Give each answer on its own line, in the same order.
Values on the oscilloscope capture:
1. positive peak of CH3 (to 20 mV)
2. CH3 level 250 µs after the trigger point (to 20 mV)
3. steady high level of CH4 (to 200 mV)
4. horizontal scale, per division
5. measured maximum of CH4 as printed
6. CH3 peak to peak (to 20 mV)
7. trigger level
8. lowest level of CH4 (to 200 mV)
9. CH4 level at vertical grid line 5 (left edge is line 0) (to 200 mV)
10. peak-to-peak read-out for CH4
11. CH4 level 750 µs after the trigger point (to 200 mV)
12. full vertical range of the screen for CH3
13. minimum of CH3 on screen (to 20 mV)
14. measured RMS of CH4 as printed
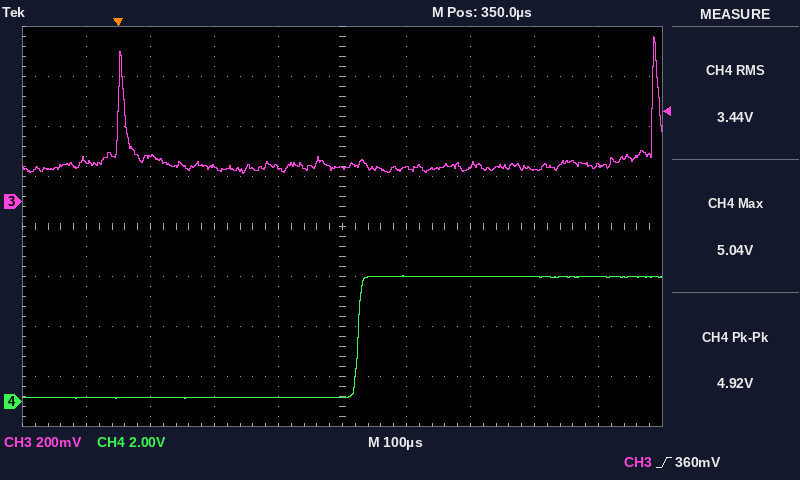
660 mV
140 mV
5.0 V
100 µs
5.04 V
540 mV
360 mV
200 mV
200 mV
4.92 V
5.0 V
1.6 V
120 mV
3.44 V
